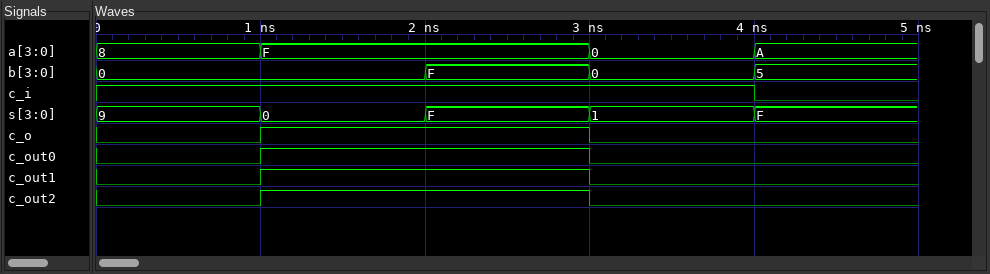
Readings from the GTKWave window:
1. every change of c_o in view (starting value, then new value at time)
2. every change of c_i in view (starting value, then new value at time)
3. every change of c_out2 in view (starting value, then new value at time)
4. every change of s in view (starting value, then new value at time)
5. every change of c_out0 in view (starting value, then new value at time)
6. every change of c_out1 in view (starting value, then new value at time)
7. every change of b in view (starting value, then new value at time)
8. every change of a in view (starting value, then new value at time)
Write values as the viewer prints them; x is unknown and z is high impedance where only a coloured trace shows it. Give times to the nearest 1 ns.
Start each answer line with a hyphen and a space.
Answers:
- 0, 1 at 1 ns, 0 at 3 ns
- 1, 0 at 4 ns
- 0, 1 at 1 ns, 0 at 3 ns
- 9, 0 at 1 ns, F at 2 ns, 1 at 3 ns, F at 4 ns
- 0, 1 at 1 ns, 0 at 3 ns
- 0, 1 at 1 ns, 0 at 3 ns
- 0, F at 2 ns, 0 at 3 ns, 5 at 4 ns
- 8, F at 1 ns, 0 at 3 ns, A at 4 ns
